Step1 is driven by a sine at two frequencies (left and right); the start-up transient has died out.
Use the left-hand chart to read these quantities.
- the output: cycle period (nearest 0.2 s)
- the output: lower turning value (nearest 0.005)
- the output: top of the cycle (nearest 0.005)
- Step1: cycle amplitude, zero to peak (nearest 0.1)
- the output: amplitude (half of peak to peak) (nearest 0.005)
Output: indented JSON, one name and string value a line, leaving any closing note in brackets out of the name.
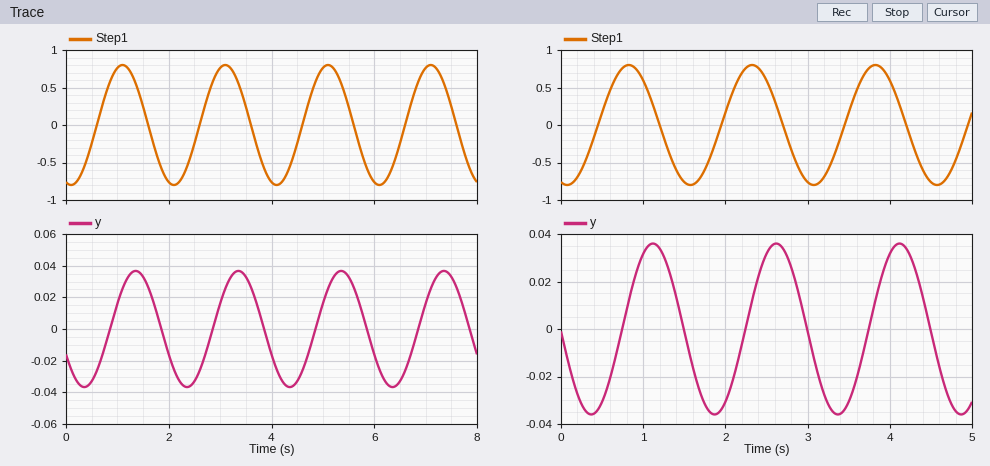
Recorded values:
{
  "the output: cycle period": "2.0 s",
  "the output: lower turning value": "-0.035",
  "the output: top of the cycle": "0.035",
  "Step1: cycle amplitude, zero to peak": "0.8",
  "the output: amplitude (half of peak to peak)": "0.035"
}
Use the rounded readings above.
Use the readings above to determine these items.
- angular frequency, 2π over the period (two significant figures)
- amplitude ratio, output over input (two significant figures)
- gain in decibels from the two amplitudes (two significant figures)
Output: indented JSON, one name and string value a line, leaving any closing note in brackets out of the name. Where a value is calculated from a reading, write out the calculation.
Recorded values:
{
  "angular frequency, 2π over the period": "2π / 2 = 3.1 rad/s",
  "amplitude ratio, output over input": "0.035 / 0.8 = 0.044",
  "gain in decibels from the two amplitudes": "20 log10(0.035 / 0.8) = -27 dB"
}
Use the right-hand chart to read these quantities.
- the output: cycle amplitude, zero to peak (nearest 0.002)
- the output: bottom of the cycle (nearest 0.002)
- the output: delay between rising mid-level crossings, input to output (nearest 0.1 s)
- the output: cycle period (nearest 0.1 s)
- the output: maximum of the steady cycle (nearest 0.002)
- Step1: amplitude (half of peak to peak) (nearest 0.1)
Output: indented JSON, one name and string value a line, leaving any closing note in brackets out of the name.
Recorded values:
{
  "the output: cycle amplitude, zero to peak": "0.036",
  "the output: bottom of the cycle": "-0.036",
  "the output: delay between rising mid-level crossings, input to output": "0.3 s",
  "the output: cycle period": "1.5 s",
  "the output: maximum of the steady cycle": "0.036",
  "Step1: amplitude (half of peak to peak)": "0.8"
}
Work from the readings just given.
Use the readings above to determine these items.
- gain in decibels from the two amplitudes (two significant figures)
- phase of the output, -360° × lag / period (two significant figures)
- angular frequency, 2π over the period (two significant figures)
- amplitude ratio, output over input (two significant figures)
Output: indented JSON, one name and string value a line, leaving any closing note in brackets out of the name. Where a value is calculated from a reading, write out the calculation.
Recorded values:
{
  "gain in decibels from the two amplitudes": "20 log10(0.036 / 0.8) = -27 dB",
  "phase of the output, -360° × lag / period": "-360 × 0.3 / 1.5 = -72°",
  "angular frequency, 2π over the period": "2π / 1.5 = 4.2 rad/s",
  "amplitude ratio, output over input": "0.036 / 0.8 = 0.045"
}
